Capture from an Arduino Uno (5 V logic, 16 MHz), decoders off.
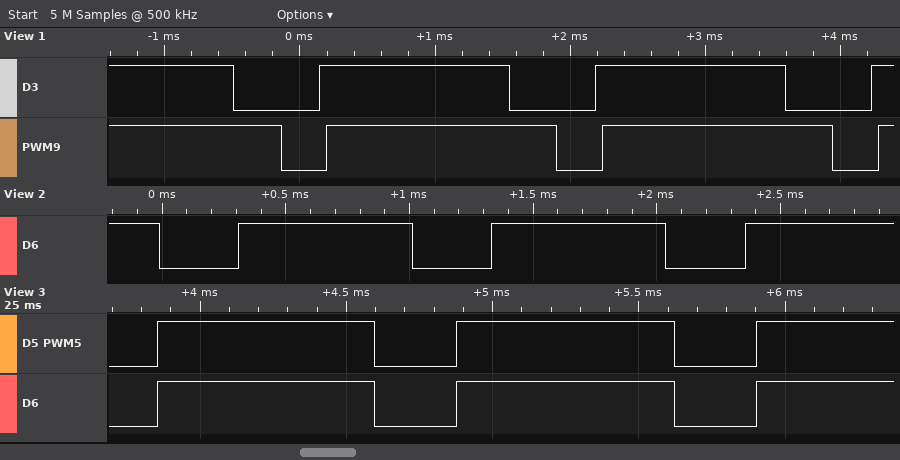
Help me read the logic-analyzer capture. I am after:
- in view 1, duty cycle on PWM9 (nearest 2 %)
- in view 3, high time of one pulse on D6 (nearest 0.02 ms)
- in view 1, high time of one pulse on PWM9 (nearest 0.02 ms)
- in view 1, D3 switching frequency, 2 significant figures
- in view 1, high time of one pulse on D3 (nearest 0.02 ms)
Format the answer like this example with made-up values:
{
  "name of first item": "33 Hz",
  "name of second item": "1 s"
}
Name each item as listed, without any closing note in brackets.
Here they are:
{
  "in view 1, duty cycle on PWM9": "84 %",
  "in view 3, high time of one pulse on D6": "0.74 ms",
  "in view 1, high time of one pulse on PWM9": "1.70 ms",
  "in view 1, D3 switching frequency, 2 significant figures": "490 Hz",
  "in view 1, high time of one pulse on D3": "1.40 ms"
}
